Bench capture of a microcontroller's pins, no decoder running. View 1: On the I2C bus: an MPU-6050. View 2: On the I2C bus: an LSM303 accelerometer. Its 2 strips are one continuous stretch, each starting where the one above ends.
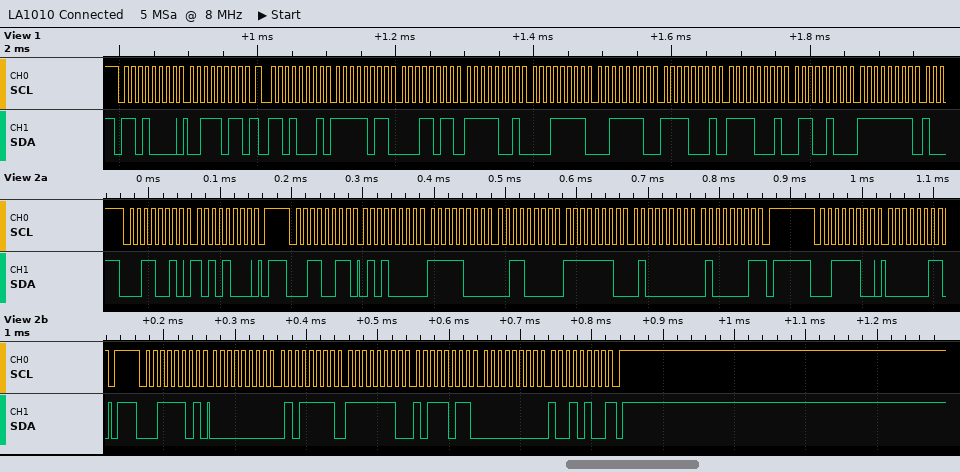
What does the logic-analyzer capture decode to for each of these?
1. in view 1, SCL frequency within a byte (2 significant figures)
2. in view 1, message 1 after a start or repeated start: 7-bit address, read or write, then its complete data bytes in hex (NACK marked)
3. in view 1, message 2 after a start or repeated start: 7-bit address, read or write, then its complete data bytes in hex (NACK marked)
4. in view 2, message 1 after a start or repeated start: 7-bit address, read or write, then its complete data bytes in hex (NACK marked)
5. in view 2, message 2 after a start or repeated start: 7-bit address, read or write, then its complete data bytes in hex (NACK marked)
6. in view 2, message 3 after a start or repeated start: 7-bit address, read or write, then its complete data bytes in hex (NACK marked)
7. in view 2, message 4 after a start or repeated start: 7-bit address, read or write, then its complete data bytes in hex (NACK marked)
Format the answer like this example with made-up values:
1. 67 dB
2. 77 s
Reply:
1. 100 kHz
2. 0x68 write: 3B
3. 0x68 read: FB 1B F9 1F 3E F1 F1 64 FF
4. 0x19 write: A8
5. 0x19 read: 50 F8 30 FE 40 41 NACK
6. 0x1E write: 03
7. 0x1E read: 00 5F FE BB 00 94 NACK
